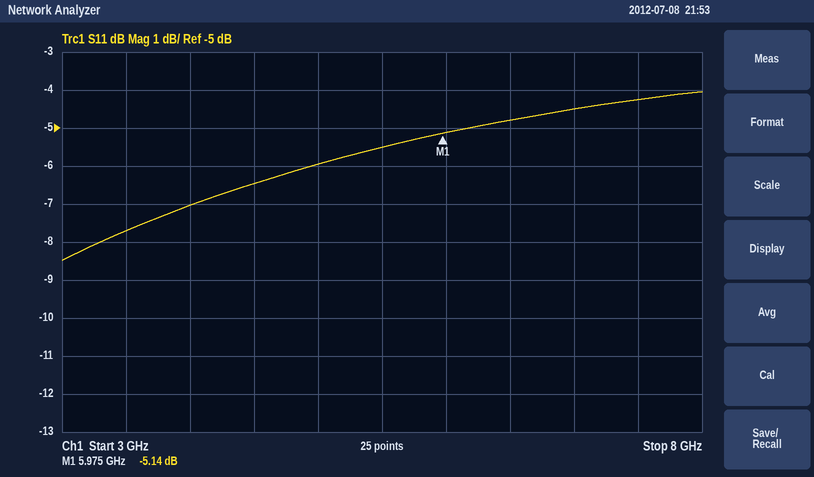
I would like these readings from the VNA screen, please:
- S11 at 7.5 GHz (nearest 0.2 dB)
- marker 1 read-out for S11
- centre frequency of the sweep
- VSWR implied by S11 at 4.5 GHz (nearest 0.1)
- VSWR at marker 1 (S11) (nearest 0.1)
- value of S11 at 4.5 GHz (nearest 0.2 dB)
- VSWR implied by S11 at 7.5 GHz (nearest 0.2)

-4.2 dB
-5.14 dB
5.5 GHz
2.8
3.5
-6.4 dB
4.2
